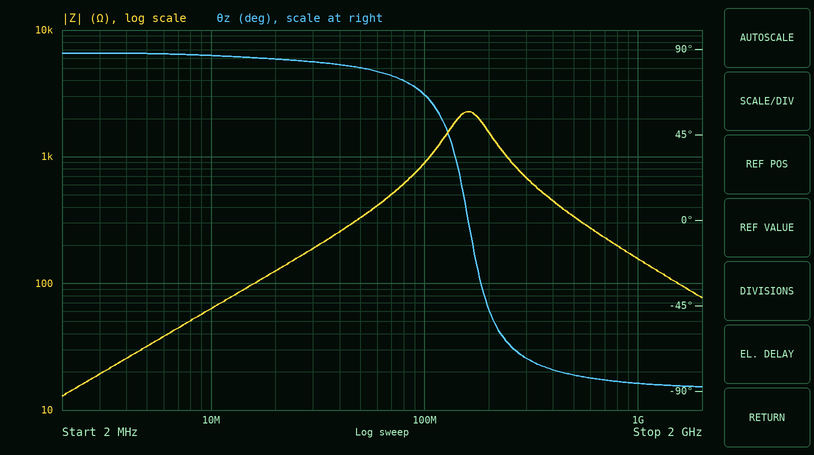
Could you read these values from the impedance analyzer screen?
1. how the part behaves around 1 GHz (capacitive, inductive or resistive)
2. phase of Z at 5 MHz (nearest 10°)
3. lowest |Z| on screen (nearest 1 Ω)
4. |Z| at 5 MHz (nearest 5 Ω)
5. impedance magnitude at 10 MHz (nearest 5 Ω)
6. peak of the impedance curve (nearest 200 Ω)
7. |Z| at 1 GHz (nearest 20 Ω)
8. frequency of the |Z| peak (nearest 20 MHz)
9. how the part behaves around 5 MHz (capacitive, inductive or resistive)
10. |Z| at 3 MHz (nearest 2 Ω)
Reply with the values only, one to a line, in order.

capacitive
90°
13 Ω
30 Ω
65 Ω
2.2 kΩ
160 Ω
160 MHz
inductive
20 Ω
